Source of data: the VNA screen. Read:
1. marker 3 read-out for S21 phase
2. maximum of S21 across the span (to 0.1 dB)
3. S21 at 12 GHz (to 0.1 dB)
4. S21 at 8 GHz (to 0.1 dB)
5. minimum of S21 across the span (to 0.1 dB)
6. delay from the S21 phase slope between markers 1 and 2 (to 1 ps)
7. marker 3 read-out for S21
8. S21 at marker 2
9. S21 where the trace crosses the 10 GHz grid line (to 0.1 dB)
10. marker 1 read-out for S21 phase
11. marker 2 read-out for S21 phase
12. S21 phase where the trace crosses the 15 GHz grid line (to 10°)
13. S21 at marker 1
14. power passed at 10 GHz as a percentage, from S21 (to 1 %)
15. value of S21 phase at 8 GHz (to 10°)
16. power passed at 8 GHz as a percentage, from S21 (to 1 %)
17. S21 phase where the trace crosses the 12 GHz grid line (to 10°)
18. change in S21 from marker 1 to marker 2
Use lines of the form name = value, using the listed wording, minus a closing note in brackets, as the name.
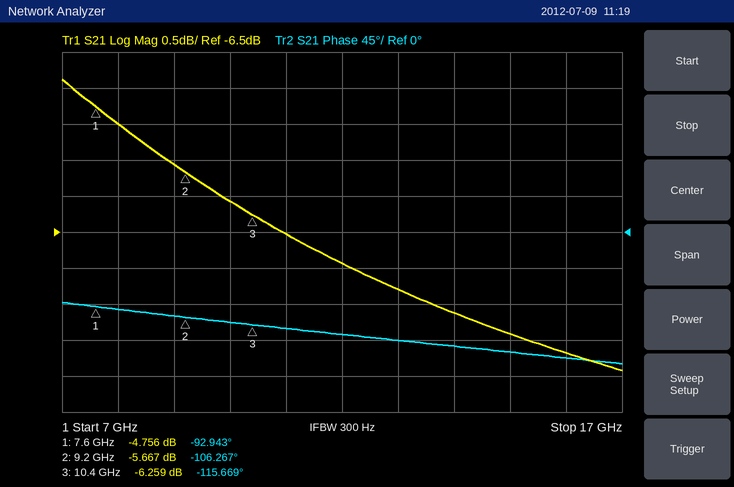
marker 3 read-out for S21 phase = -115.669°
maximum of S21 across the span = -4.4 dB
S21 at 12 GHz = -6.9 dB
S21 at 8 GHz = -5.0 dB
minimum of S21 across the span = -8.4 dB
delay from the S21 phase slope between markers 1 and 2 = 23 ps
marker 3 read-out for S21 = -6.259 dB
S21 at marker 2 = -5.667 dB
S21 where the trace crosses the 10 GHz grid line = -6.1 dB
marker 1 read-out for S21 phase = -92.943°
marker 2 read-out for S21 phase = -106.267°
S21 phase where the trace crosses the 15 GHz grid line = -150°
S21 at marker 1 = -4.756 dB
power passed at 10 GHz as a percentage, from S21 = 25 %
value of S21 phase at 8 GHz = -100°
power passed at 8 GHz as a percentage, from S21 = 32 %
S21 phase where the trace crosses the 12 GHz grid line = -130°
change in S21 from marker 1 to marker 2 = -0.911 dB
